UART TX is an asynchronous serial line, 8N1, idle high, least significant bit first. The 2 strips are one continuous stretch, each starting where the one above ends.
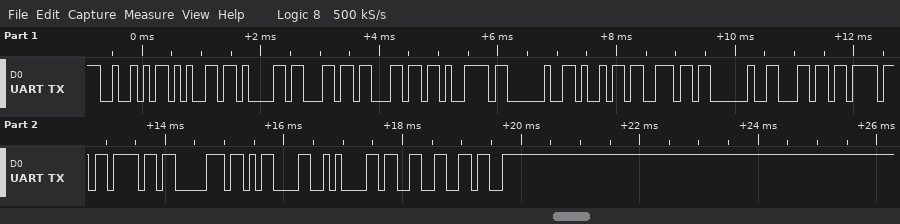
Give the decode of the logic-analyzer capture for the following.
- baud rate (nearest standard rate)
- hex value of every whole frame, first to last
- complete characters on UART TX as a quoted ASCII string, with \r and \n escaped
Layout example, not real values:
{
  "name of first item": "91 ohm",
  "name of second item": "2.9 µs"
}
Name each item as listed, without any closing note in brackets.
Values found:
{
  "baud rate": "9600 baud",
  "hex value of every whole frame, first to last": "0x52 0x65 0x61 0x6C 0x6C 0x79 0x20 0x69 0x6E 0x20 0x6C 0x6F 0x6F 0x70 0x0D 0x0A 0x33 0x36",
  "complete characters on UART TX as a quoted ASCII string, with \\r and \\n escaped": "\"Really in loop\\r\\n36\""
}
